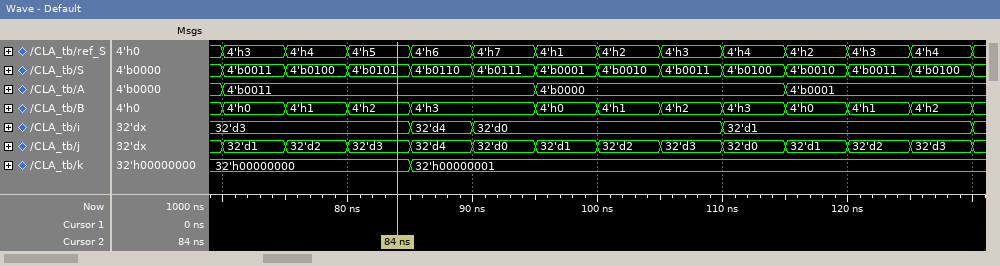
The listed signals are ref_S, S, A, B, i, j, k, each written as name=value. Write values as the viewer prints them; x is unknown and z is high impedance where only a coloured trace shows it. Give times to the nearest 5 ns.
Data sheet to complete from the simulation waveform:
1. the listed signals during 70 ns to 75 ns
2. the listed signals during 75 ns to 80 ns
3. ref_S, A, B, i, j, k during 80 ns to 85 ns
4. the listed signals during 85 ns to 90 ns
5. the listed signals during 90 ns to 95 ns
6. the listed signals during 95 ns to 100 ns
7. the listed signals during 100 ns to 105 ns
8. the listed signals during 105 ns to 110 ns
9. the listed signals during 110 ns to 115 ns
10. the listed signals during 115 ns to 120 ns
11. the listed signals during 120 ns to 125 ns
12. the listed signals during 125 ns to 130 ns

ref_S=4'h3, S=4'b0011, A=4'b0011, B=4'h0, i=32'd3, j=32'd1, k=32'h00000000
ref_S=4'h4, S=4'b0100, A=4'b0011, B=4'h1, i=32'd3, j=32'd2, k=32'h00000000
ref_S=4'h5, A=4'b0011, B=4'h2, i=32'd3, j=32'd3, k=32'h00000000
ref_S=4'h6, S=4'b0110, A=4'b0011, B=4'h3, i=32'd4, j=32'd4, k=32'h00000001
ref_S=4'h7, S=4'b0111, A=4'b0011, B=4'h3, i=32'd0, j=32'd0, k=32'h00000001
ref_S=4'h1, S=4'b0001, A=4'b0000, B=4'h0, i=32'd0, j=32'd1, k=32'h00000001
ref_S=4'h2, S=4'b0010, A=4'b0000, B=4'h1, i=32'd0, j=32'd2, k=32'h00000001
ref_S=4'h3, S=4'b0011, A=4'b0000, B=4'h2, i=32'd0, j=32'd3, k=32'h00000001
ref_S=4'h4, S=4'b0100, A=4'b0000, B=4'h3, i=32'd1, j=32'd0, k=32'h00000001
ref_S=4'h2, S=4'b0010, A=4'b0001, B=4'h0, i=32'd1, j=32'd1, k=32'h00000001
ref_S=4'h3, S=4'b0011, A=4'b0001, B=4'h1, i=32'd1, j=32'd2, k=32'h00000001
ref_S=4'h4, S=4'b0100, A=4'b0001, B=4'h2, i=32'd1, j=32'd3, k=32'h00000001
